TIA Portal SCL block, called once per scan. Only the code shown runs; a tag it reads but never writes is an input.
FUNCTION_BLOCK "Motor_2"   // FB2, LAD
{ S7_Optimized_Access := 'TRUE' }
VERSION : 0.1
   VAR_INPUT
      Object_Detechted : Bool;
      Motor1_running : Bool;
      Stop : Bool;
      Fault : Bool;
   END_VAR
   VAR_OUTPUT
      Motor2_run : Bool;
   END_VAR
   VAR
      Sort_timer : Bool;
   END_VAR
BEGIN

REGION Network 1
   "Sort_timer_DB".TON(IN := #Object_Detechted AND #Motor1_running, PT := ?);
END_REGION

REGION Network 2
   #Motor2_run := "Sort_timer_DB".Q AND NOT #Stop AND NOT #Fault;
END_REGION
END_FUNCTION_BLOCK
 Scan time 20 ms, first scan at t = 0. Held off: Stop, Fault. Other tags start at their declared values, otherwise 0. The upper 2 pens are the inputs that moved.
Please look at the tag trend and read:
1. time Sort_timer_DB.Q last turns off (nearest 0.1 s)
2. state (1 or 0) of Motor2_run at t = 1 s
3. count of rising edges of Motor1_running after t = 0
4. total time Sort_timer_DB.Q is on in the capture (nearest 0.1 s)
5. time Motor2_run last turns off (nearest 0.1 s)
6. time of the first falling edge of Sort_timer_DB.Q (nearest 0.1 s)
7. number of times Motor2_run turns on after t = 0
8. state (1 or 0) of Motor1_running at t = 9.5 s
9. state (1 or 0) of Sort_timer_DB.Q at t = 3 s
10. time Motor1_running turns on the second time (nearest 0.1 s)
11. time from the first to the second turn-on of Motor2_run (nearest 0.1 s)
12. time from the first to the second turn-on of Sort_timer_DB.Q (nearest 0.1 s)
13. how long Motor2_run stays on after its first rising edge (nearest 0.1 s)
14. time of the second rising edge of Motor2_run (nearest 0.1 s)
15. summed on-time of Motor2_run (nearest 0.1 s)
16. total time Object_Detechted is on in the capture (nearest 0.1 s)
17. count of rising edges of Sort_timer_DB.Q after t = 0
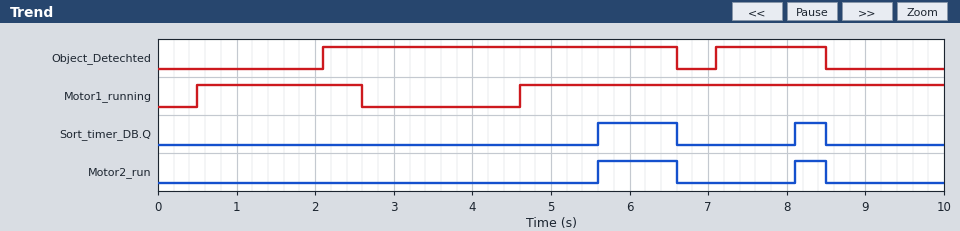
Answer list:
8.5 s
0
2
1.4 s
8.5 s
6.6 s
2
1
0
4.6 s
2.5 s
2.5 s
1.0 s
8.1 s
1.4 s
5.9 s
2
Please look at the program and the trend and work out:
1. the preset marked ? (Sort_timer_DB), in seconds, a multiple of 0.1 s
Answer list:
1.0 s
